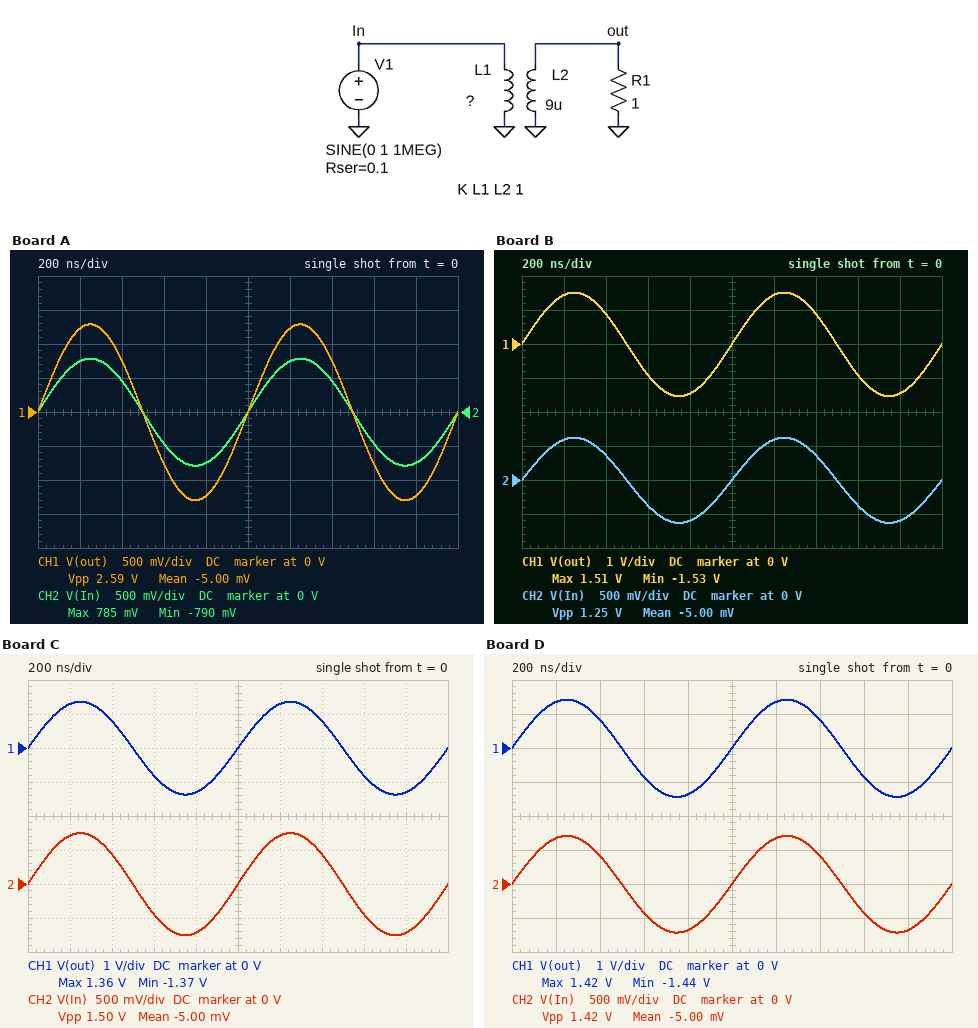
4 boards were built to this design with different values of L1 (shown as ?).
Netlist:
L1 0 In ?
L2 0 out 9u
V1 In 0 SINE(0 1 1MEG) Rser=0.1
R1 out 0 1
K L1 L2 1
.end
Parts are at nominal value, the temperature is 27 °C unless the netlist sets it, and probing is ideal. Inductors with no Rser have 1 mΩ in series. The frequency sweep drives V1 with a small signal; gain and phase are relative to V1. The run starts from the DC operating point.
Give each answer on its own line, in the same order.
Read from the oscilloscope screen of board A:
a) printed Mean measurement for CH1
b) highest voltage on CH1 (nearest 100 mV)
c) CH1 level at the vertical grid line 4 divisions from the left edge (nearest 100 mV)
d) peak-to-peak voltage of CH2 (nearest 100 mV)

-5.00 mV
1.3 V
-1.2 V
1.6 V
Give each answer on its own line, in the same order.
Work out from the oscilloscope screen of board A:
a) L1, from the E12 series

3.3 µH
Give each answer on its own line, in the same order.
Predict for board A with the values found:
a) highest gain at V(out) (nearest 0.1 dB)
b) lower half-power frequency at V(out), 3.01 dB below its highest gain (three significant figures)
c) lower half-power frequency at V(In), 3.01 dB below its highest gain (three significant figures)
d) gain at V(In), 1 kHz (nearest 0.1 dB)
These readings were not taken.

2.2 dB
3.82 kHz
3.82 kHz
-14.0 dB
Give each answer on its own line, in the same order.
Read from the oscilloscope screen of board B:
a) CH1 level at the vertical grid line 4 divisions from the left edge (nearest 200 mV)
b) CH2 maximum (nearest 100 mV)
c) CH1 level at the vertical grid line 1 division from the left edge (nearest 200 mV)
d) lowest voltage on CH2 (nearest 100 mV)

-1.4 V
600 mV
1.4 V
-600 mV
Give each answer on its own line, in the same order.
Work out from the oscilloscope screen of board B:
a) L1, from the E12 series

1.5 µH
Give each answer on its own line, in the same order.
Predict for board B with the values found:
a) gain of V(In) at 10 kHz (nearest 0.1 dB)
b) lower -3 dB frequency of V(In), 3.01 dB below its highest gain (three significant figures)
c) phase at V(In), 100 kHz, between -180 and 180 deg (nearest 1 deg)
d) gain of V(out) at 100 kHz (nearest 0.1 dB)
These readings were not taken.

-5.7 dB
6.67 kHz
4 deg
3.6 dB
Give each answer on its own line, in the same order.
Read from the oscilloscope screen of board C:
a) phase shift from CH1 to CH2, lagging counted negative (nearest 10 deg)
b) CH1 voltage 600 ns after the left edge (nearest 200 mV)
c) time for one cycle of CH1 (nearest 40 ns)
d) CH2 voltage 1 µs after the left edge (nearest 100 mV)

0 deg
-800 mV
1.00 µs
0 V
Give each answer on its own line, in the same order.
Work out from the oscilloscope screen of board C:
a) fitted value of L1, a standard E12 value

2.7 µH
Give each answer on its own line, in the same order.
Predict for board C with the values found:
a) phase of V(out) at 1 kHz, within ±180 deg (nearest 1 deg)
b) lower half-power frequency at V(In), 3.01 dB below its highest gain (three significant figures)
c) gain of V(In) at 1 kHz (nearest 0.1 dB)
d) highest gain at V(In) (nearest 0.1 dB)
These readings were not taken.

77 deg
4.45 kHz
-15.7 dB
-2.5 dB
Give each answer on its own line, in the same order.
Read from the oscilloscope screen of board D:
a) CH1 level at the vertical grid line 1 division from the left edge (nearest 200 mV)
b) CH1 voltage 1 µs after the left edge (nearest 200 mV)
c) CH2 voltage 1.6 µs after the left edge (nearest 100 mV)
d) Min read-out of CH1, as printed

1.4 V
0 V
-400 mV
-1.44 V
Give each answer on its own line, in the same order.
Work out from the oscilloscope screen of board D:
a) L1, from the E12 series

2.2 µH
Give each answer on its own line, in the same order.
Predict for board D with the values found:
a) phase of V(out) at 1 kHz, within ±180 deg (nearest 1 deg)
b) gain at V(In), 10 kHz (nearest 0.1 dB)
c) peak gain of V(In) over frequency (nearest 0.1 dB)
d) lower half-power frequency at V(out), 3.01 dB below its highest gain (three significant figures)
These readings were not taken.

79 deg
-4.0 dB
-3.0 dB
5.17 kHz
